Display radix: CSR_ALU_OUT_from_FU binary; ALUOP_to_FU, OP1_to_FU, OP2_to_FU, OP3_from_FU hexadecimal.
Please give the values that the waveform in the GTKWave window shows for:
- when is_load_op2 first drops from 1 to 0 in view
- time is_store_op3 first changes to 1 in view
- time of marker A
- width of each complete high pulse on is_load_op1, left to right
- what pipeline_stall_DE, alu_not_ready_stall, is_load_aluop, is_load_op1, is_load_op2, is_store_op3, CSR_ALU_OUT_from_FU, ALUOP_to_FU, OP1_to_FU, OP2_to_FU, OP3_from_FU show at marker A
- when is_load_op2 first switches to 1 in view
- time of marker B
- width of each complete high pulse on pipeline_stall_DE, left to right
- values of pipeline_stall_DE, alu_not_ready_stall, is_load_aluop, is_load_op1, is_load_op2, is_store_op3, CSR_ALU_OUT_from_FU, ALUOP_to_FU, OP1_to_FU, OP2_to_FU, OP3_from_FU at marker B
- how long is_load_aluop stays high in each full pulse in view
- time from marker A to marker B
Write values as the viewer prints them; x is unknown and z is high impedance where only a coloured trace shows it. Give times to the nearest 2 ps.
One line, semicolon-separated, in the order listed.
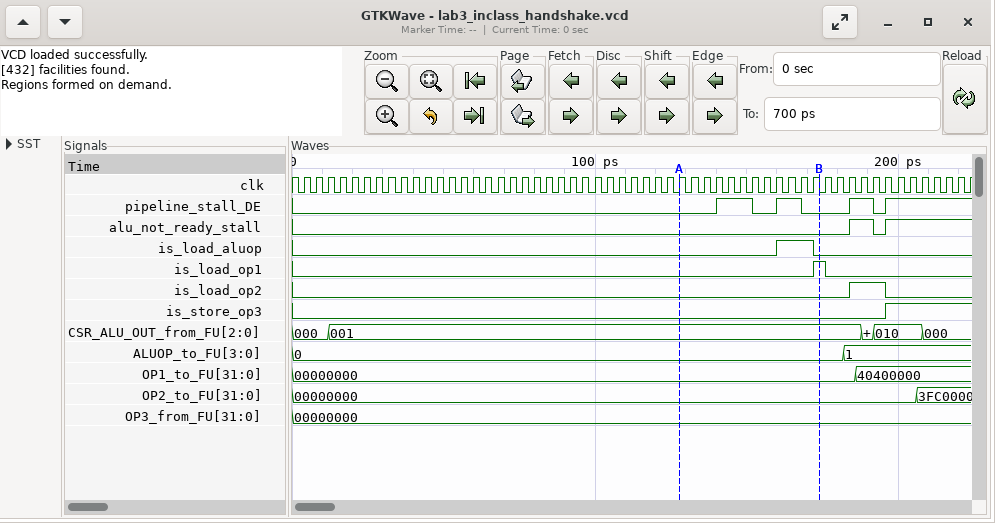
196 ps; 196 ps; 128 ps; 4 ps; pipeline_stall_DE=0, alu_not_ready_stall=0, is_load_aluop=0, is_load_op1=0, is_load_op2=0, is_store_op3=0, CSR_ALU_OUT_from_FU=001, ALUOP_to_FU=0, OP1_to_FU=00000000, OP2_to_FU=00000000, OP3_from_FU=00000000; 184 ps; 174 ps; 12 ps, 8 ps, 8 ps; pipeline_stall_DE=0, alu_not_ready_stall=0, is_load_aluop=0, is_load_op1=1, is_load_op2=0, is_store_op3=0, CSR_ALU_OUT_from_FU=001, ALUOP_to_FU=0, OP1_to_FU=00000000, OP2_to_FU=00000000, OP3_from_FU=00000000; 12 ps; 46 ps
